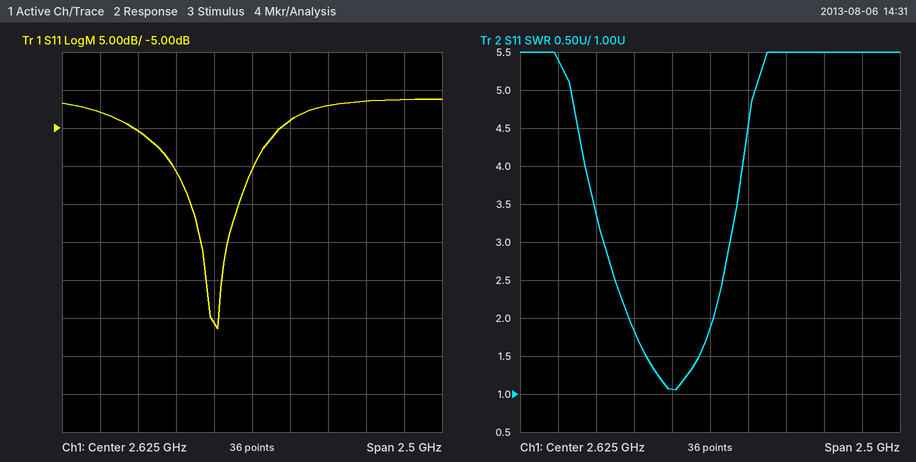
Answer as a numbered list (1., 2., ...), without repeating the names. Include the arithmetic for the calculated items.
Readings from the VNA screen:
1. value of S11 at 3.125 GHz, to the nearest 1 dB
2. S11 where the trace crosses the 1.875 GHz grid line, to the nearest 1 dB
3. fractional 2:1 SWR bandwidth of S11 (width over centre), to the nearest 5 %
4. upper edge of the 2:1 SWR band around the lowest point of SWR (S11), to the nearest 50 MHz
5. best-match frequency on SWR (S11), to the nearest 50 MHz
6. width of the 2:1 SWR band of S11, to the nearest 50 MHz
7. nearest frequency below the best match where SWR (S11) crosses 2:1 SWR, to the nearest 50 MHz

1. -2 dB
2. -5 dB
3. 550 MHz / 2.375 GHz ≈ 23.2 %, so 25 % to the nearest 5 %
4. 2.65 GHz
5. 2.40 GHz
6. 2.65 GHz − 2.10 GHz = 550 MHz
7. 2.10 GHz
